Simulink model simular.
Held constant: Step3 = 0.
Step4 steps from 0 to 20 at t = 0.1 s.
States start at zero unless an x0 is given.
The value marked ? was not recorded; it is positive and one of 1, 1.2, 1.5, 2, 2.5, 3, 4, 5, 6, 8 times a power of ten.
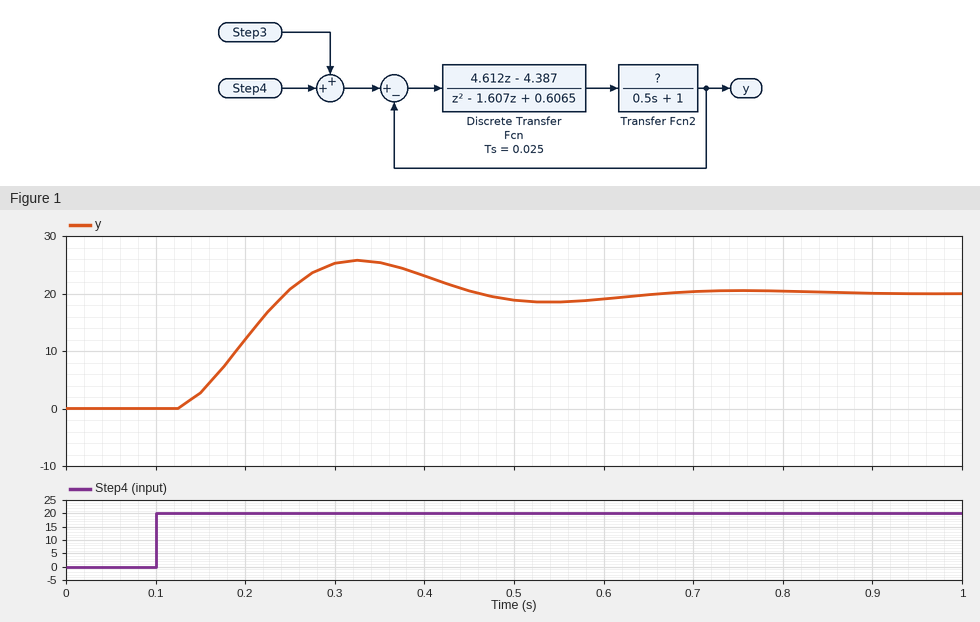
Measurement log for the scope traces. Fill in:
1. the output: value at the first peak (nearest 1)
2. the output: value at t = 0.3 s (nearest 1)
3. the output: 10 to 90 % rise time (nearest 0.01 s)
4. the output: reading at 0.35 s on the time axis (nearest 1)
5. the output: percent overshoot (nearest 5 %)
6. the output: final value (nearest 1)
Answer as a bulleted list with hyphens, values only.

- 26
- 25
- 0.09 s
- 25
- 30 %
- 20
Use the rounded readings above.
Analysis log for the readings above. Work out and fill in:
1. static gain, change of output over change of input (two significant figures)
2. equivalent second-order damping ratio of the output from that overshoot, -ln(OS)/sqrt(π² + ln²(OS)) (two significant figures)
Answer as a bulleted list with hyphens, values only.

- 1.0
- 0.36
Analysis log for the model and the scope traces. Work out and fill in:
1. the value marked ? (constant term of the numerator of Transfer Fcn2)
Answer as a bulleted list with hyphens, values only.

- 0.6
